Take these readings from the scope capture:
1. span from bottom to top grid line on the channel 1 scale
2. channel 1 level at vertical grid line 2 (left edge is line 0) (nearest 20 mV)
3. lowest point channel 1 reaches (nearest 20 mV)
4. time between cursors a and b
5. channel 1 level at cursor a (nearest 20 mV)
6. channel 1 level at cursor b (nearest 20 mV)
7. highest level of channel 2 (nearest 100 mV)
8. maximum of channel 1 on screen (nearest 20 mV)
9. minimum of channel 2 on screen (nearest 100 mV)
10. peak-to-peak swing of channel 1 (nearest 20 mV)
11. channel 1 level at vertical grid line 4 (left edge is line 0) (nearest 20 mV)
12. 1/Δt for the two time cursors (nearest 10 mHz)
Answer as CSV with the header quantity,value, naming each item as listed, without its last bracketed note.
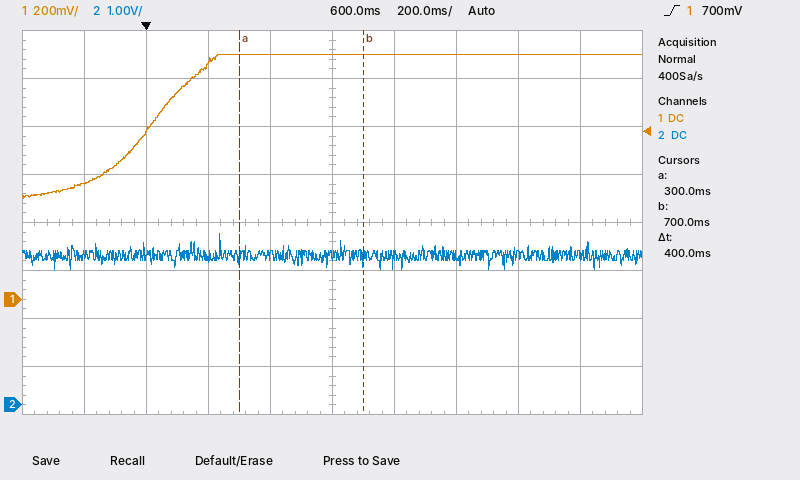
quantity,value
span from bottom to top grid line on the channel 1 scale,1.6 V
channel 1 level at vertical grid line 2 (left edge is line 0),700 mV
lowest point channel 1 reaches,420 mV
time between cursors a and b,400 ms
channel 1 level at cursor a,1.02 V
channel 1 level at cursor b,1.02 V
highest level of channel 2,3.6 V
maximum of channel 1 on screen,1.02 V
minimum of channel 2 on screen,2.8 V
peak-to-peak swing of channel 1,600 mV
channel 1 level at vertical grid line 4 (left edge is line 0),1.02 V
1/Δt for the two time cursors,2.50 Hz
